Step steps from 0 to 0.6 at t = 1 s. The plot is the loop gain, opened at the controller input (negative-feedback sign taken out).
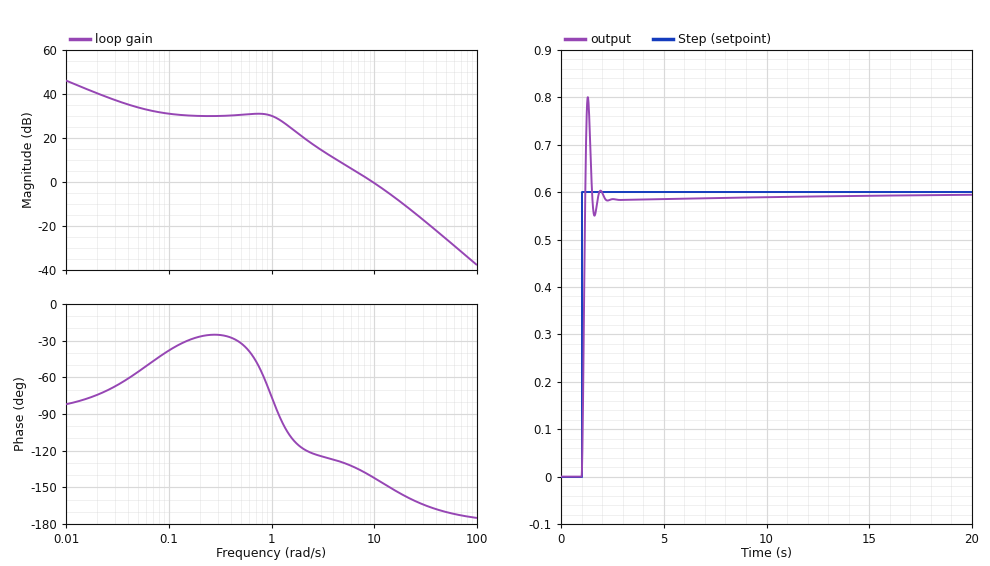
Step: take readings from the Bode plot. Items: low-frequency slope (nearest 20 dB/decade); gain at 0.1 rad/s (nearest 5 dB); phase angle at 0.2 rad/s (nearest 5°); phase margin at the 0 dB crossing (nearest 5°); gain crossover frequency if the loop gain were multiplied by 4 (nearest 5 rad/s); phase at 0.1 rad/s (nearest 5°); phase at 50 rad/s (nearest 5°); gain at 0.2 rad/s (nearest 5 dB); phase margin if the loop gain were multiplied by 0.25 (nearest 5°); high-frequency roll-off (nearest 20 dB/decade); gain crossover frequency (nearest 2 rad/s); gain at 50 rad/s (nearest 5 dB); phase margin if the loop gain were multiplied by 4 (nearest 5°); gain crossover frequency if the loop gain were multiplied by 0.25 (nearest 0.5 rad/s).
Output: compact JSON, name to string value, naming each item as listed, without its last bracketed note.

{"low-frequency slope": "-20 dB/decade", "gain at 0.1 rad/s": "30 dB", "phase angle at 0.2 rad/s": "-25°", "phase margin at the 0 dB crossing": "40°", "gain crossover frequency if the loop gain were multiplied by 4": "20 rad/s", "phase at 0.1 rad/s": "-40°", "phase at 50 rad/s": "-170°", "gain at 0.2 rad/s": "30 dB", "phase margin if the loop gain were multiplied by 0.25": "55°", "high-frequency roll-off": "-40 dB/decade", "gain crossover frequency": "10 rad/s", "gain at 50 rad/s": "-25 dB", "phase margin if the loop gain were multiplied by 4": "20°", "gain crossover frequency if the loop gain were multiplied by 0.25": "3.5 rad/s"}
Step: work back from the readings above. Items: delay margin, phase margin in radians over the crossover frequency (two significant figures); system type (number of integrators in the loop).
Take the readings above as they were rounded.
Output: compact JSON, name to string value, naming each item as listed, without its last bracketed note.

{"delay margin, phase margin in radians over the crossover frequency": "0.070 s", "system type": "1"}
